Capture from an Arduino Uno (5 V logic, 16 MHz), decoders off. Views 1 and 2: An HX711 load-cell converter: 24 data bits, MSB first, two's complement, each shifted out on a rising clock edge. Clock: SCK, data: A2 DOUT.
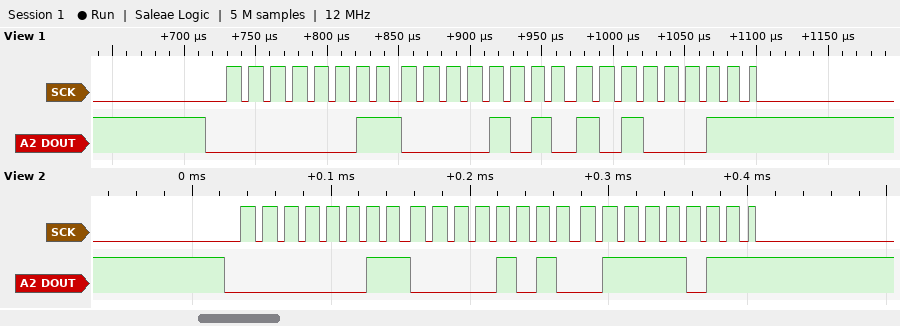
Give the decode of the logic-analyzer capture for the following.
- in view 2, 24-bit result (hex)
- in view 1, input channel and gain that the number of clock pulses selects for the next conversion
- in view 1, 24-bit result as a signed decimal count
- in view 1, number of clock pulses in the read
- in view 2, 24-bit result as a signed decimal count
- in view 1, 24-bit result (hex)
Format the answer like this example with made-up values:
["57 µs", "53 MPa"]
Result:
["0x030A7B", "channel A, gain 128", "199331", "25", "199291", "0x030AA3"]
